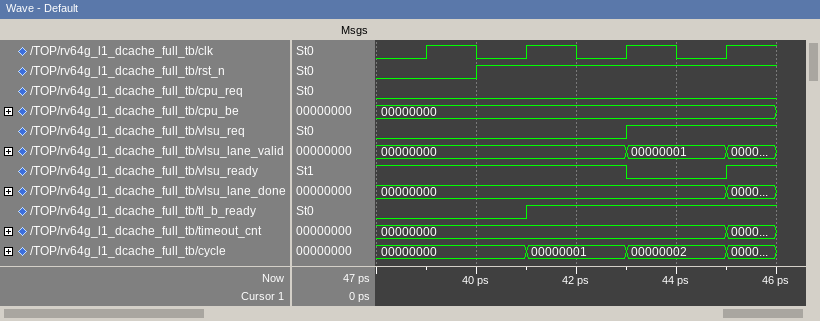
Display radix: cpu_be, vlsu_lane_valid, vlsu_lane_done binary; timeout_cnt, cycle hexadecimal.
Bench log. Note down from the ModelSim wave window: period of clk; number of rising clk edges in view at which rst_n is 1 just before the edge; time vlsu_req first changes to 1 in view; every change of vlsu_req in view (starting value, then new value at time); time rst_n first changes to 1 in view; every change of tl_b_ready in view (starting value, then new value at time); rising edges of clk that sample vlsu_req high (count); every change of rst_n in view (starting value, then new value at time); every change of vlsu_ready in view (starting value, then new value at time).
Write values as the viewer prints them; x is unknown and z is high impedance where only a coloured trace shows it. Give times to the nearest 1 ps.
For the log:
2 ps
3
43 ps
0, 1 at 43 ps
40 ps
0, 1 at 41 ps
1
0, 1 at 40 ps
1, 0 at 43 ps, 1 at 45 ps
